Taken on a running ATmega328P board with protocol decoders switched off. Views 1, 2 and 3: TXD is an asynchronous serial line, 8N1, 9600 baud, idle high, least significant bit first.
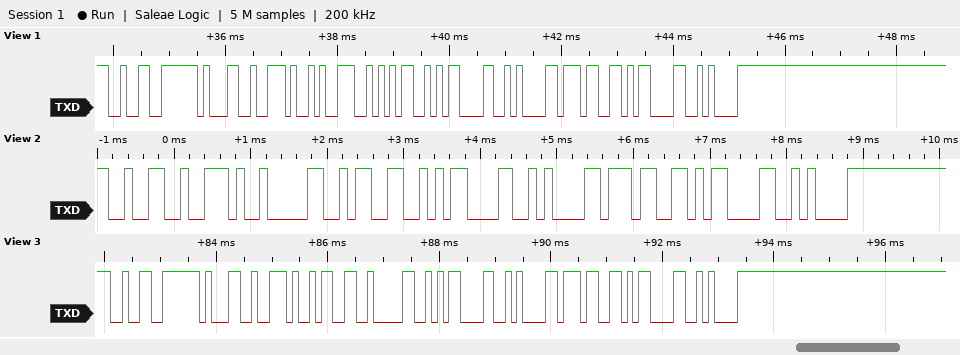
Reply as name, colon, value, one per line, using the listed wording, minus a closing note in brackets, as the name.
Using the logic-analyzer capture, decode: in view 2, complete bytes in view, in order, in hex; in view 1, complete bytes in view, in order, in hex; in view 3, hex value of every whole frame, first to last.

in view 2, complete bytes in view, in order, in hex: 32 2E 30 33 0D 0A 37 0D 0A
in view 1, complete bytes in view, in order, in hex: 32 31 2E 39 35 0D 0A 37 0D 0A
in view 3, hex value of every whole frame, first to last: 32 31 2E 33 30 0D 0A 37 0D 0A
